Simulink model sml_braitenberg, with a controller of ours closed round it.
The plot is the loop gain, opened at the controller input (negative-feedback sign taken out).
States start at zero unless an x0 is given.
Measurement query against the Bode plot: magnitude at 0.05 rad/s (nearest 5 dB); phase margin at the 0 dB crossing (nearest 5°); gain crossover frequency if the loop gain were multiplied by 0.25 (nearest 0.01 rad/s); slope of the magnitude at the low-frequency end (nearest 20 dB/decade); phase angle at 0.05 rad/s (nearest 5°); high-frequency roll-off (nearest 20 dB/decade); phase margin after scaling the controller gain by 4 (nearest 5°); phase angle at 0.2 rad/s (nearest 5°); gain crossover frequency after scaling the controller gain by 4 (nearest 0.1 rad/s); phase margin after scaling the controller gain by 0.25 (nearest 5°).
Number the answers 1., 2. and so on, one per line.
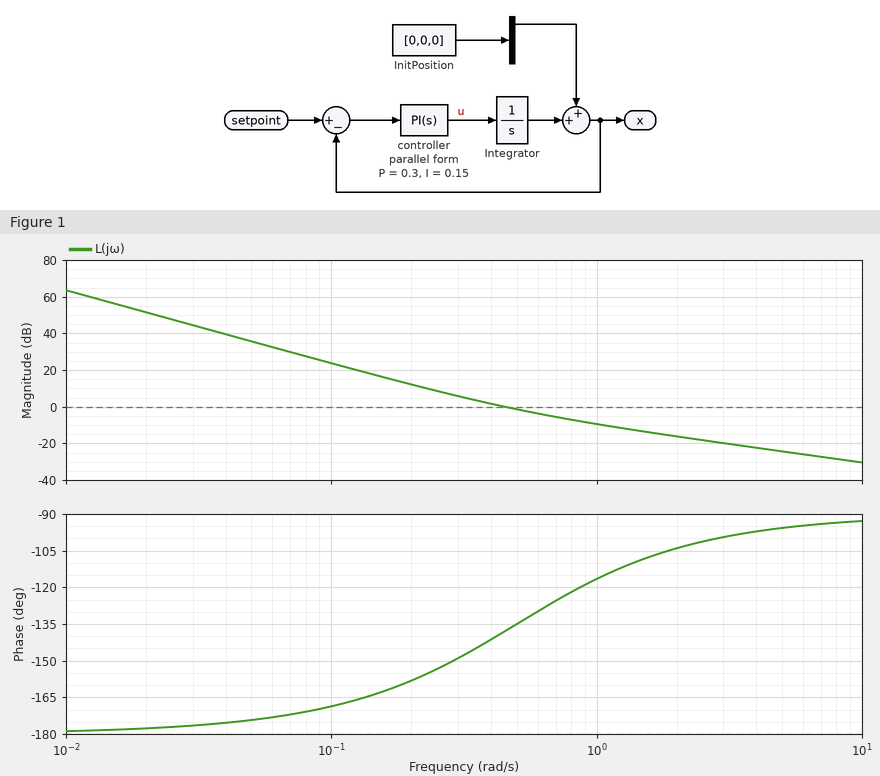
1. 35 dB
2. 40°
3. 0.20 rad/s
4. -40 dB/decade
5. -175°
6. -20 dB/decade
7. 70°
8. -160°
9. 1.3 rad/s
10. 20°
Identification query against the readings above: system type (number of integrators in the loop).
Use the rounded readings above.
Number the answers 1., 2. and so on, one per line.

1. 2
